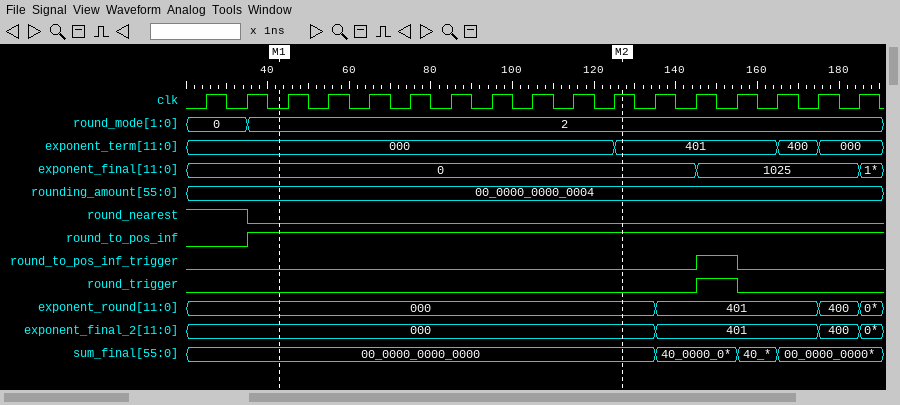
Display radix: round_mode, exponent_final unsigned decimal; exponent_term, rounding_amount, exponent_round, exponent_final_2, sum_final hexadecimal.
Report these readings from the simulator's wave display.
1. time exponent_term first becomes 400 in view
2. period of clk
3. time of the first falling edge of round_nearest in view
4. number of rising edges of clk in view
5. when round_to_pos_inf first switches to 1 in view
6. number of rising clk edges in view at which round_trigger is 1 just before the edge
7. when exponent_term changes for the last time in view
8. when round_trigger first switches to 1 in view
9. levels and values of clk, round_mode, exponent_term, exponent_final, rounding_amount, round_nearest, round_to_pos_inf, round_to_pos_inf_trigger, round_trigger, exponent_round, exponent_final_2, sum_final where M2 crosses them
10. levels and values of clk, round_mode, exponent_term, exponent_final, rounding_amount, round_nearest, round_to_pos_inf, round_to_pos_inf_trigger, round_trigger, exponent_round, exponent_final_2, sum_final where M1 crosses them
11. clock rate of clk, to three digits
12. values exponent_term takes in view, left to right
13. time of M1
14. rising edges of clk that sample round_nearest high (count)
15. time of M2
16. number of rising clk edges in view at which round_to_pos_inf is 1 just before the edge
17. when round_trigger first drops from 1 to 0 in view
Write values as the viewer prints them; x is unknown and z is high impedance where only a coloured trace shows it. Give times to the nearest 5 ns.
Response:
165 ns
10 ns
35 ns
17
35 ns
1
175 ns
145 ns
clk=1, round_mode=2, exponent_term=401, exponent_final=0, rounding_amount=00_0000_0000_0004, round_nearest=0, round_to_pos_inf=1, round_to_pos_inf_trigger=0, round_trigger=0, exponent_round=000, exponent_final_2=000, sum_final=00_0000_0000_0000
clk=0, round_mode=2, exponent_term=000, exponent_final=0, rounding_amount=00_0000_0000_0004, round_nearest=0, round_to_pos_inf=1, round_to_pos_inf_trigger=0, round_trigger=0, exponent_round=000, exponent_final_2=000, sum_final=00_0000_0000_0000
100 MHz
000, 401, 400, 000
45 ns
2
125 ns
15
155 ns
